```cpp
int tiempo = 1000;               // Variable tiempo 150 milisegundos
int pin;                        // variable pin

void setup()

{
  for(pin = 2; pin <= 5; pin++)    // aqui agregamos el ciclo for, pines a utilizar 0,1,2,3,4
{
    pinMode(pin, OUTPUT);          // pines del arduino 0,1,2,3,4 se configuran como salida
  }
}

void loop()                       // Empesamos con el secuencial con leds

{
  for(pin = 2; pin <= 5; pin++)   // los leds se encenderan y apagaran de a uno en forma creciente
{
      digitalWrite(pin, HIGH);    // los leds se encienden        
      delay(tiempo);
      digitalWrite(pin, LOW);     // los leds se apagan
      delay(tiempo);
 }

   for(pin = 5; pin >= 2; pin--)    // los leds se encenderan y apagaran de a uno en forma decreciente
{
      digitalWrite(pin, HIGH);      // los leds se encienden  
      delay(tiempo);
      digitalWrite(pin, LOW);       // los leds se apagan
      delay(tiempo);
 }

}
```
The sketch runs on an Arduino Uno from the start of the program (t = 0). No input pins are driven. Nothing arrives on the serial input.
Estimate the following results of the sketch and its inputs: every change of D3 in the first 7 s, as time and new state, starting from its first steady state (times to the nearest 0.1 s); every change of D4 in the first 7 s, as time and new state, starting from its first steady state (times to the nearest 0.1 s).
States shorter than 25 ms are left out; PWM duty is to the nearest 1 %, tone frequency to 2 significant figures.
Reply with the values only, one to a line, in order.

0 s low; 2 s high; 3 s low
0 s low; 4 s high; 5 s low
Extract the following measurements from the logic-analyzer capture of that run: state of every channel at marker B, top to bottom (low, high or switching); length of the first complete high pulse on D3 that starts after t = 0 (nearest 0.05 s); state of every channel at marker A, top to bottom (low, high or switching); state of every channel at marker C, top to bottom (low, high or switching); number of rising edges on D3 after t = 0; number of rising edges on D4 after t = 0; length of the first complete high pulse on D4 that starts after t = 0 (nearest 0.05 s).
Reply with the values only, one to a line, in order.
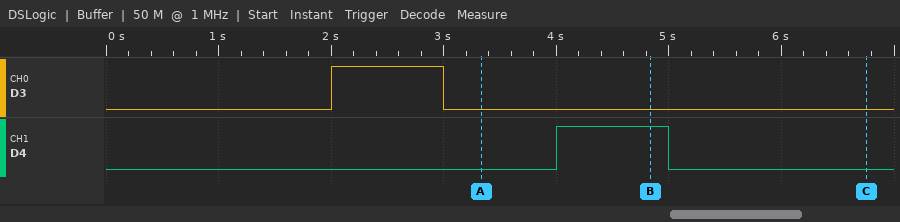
D3 low, D4 high
1.00 s
D3 low, D4 low
D3 low, D4 low
1
1
1.00 s
